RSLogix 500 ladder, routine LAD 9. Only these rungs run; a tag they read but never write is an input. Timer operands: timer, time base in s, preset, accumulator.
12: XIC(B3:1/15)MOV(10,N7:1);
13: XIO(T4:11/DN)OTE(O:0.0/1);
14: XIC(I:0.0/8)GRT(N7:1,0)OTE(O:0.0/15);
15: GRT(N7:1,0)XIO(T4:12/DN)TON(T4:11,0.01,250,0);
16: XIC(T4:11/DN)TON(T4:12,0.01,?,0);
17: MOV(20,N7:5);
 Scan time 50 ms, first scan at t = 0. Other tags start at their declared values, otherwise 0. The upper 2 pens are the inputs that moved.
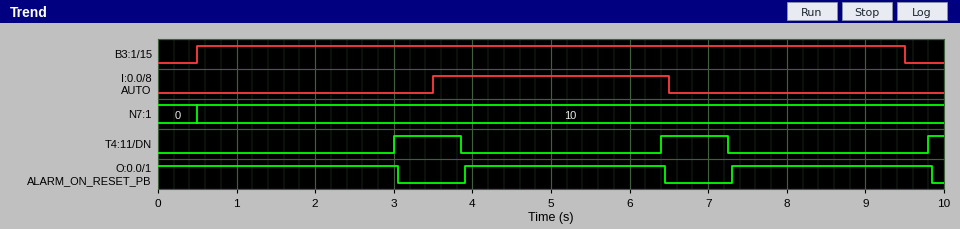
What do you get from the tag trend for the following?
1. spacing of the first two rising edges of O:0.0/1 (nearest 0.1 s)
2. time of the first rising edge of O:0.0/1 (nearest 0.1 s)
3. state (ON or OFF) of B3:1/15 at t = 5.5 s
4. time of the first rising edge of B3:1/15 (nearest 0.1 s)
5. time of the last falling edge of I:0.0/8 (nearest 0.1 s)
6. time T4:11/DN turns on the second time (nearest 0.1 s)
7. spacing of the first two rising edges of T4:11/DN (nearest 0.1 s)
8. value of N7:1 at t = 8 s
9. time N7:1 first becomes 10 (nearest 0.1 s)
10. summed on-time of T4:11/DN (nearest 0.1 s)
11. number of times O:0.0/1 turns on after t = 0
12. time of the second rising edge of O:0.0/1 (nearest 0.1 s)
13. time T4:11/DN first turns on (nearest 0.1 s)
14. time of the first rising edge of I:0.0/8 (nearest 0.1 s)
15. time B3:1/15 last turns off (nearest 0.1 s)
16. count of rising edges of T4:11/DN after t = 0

3.4 s
3.9 s
ON
0.5 s
6.5 s
6.4 s
3.4 s
10
0.5 s
1.9 s
2
7.3 s
3.0 s
3.5 s
9.5 s
3
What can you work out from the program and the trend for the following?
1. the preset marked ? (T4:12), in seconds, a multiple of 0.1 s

0.8 s
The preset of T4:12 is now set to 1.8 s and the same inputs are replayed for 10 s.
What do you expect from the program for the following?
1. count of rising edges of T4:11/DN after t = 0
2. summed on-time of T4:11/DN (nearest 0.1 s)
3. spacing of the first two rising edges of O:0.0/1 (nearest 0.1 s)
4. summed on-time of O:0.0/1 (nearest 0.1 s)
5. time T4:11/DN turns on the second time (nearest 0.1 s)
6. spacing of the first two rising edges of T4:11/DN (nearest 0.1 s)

2
3.7 s
4.4 s
6.3 s
7.4 s
4.4 s
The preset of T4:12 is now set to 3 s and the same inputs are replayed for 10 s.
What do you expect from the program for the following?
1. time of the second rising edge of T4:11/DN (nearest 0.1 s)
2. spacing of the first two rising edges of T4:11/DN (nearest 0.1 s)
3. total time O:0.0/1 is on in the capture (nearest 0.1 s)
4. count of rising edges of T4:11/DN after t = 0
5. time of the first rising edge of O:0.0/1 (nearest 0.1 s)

8.6 s
5.6 s
5.6 s
2
6.1 s
